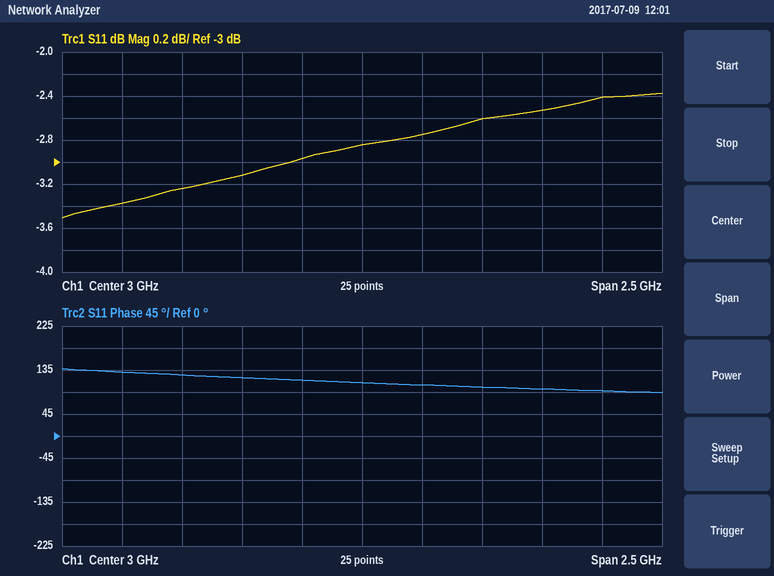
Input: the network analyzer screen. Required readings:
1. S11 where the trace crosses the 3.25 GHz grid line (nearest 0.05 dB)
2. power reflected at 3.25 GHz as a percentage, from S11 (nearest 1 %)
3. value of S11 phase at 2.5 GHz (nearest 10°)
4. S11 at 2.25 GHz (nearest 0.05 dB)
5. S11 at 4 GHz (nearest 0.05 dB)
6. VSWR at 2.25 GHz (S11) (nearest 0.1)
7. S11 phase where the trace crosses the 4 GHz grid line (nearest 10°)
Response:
-2.75 dB
53 %
120°
-3.25 dB
-2.40 dB
5.4
90°
